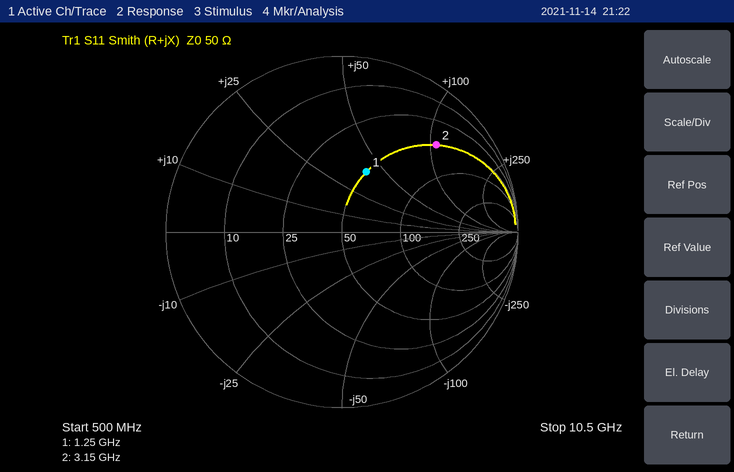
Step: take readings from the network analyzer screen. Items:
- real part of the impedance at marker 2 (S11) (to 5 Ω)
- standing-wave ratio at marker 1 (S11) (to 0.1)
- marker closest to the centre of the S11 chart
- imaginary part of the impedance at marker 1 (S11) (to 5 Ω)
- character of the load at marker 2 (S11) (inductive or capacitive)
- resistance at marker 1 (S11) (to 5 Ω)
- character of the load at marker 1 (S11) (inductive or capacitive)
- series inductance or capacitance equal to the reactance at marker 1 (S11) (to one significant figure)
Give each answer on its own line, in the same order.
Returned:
50 Ω
2.2
marker 1
+40 Ω
inductive
50 Ω
inductive
5 nH
